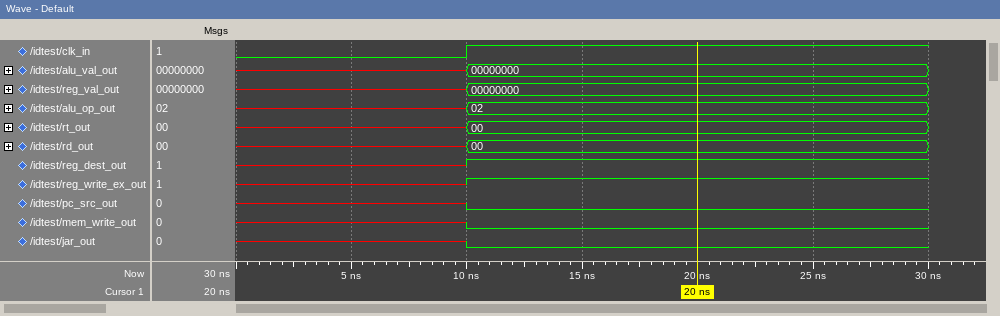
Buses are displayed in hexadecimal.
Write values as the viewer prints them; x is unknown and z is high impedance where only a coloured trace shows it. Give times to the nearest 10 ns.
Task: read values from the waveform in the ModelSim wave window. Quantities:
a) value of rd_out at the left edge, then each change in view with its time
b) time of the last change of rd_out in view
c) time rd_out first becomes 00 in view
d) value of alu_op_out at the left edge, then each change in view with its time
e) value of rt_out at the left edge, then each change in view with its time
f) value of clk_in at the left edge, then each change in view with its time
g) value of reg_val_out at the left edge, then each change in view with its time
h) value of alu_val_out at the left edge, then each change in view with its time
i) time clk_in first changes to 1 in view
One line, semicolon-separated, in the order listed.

x, 00 at 10 ns; 10 ns; 10 ns; x, 02 at 10 ns; x, 00 at 10 ns; 0, 1 at 10 ns; x, 00000000 at 10 ns; x, 00000000 at 10 ns; 10 ns
